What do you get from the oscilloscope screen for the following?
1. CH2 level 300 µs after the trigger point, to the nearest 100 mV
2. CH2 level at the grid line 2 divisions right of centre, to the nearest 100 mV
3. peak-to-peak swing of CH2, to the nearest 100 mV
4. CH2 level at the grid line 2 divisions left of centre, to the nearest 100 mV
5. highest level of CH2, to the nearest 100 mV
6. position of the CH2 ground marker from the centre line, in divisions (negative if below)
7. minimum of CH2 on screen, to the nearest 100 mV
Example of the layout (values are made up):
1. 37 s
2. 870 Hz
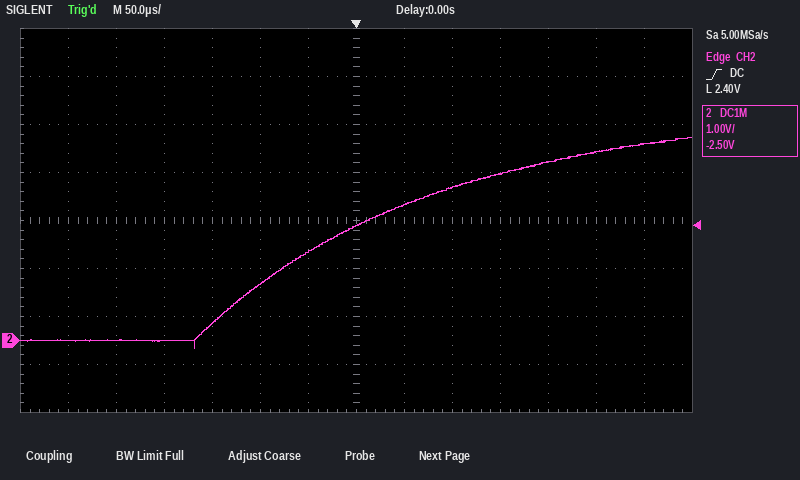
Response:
1. 4.1 V
2. 3.2 V
3. 4.4 V
4. 1.2 V
5. 4.2 V
6. -2.5 div
7. -200 mV
